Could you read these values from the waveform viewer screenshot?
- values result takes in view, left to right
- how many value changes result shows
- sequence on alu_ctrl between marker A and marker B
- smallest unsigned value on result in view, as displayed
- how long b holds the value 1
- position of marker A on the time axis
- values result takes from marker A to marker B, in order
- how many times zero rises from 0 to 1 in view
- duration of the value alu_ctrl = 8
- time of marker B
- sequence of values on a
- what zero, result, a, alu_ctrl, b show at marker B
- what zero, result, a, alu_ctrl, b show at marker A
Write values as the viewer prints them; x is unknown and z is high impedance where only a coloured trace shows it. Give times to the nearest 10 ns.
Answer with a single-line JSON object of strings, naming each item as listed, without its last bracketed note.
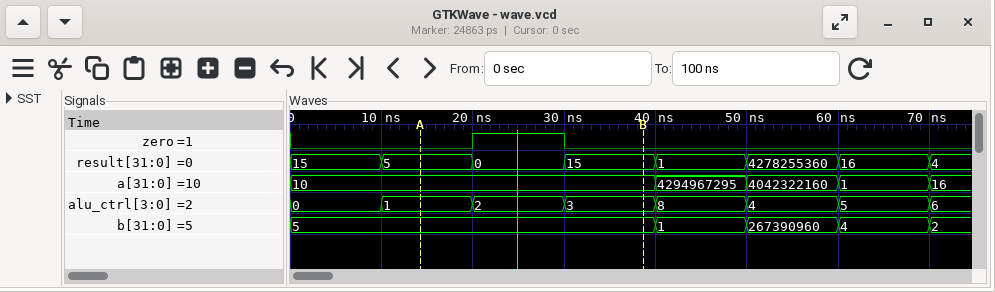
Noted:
{"values result takes in view, left to right": "15, 5, 0, 15, 1, 4278255360, 16, 4", "how many value changes result shows": "7", "sequence on alu_ctrl between marker A and marker B": "1, 2, 3", "smallest unsigned value on result in view, as displayed": "0", "how long b holds the value 1": "10 ns", "position of marker A on the time axis": "10 ns", "values result takes from marker A to marker B, in order": "5, 0, 15", "how many times zero rises from 0 to 1 in view": "1", "duration of the value alu_ctrl = 8": "10 ns", "time of marker B": "40 ns", "sequence of values on a": "10, 4294967295, 4042322160, 1, 16", "what zero, result, a, alu_ctrl, b show at marker B": "zero=0, result=15, a=10, alu_ctrl=3, b=5", "what zero, result, a, alu_ctrl, b show at marker A": "zero=0, result=5, a=10, alu_ctrl=1, b=5"}
